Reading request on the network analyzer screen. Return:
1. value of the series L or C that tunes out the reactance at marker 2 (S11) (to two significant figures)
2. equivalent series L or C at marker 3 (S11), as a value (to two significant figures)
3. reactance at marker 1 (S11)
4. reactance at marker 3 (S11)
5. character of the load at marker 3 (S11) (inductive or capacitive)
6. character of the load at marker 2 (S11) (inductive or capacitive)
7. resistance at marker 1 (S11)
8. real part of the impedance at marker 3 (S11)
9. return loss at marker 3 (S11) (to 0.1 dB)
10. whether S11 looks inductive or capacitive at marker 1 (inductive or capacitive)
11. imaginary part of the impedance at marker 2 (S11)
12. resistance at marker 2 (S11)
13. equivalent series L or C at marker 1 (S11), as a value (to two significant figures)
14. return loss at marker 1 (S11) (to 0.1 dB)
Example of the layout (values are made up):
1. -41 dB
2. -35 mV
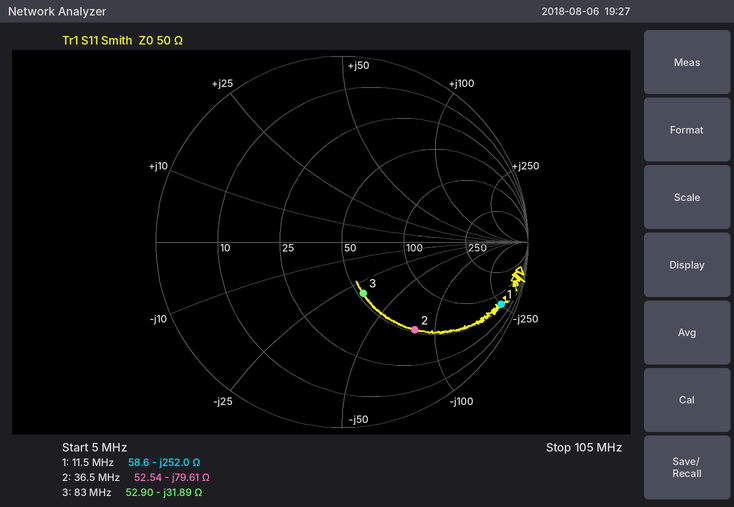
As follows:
1. 350 nH
2. 60 pF
3. -252.0 Ω
4. -31.89 Ω
5. capacitive
6. capacitive
7. 58.6 Ω
8. 52.90 Ω
9. 10.5 dB
10. capacitive
11. -79.61 Ω
12. 52.54 Ω
13. 55 pF
14. 0.7 dB
